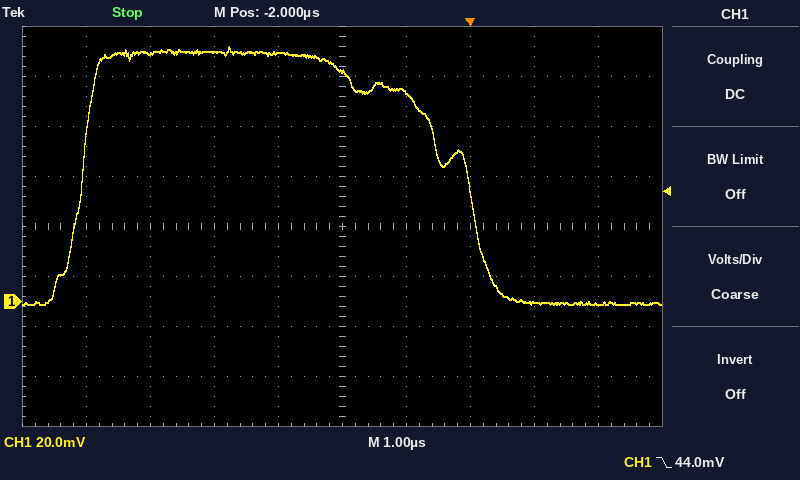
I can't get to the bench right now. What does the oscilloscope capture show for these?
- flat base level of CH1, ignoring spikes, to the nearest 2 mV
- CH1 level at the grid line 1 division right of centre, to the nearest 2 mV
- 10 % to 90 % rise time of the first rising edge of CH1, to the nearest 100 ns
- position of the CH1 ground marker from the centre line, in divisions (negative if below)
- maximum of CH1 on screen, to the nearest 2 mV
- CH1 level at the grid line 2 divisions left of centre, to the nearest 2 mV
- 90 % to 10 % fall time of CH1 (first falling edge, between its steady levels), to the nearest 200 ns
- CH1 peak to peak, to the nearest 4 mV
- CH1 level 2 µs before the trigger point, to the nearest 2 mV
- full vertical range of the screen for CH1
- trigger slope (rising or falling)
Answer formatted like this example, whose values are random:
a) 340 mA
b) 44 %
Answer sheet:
a) 0 mV
b) 84 mV
c) 600 ns
d) -1.5 div
e) 102 mV
f) 100 mV
g) 2.2 µs
h) 104 mV
i) 92 mV
j) 160 mV
k) falling
